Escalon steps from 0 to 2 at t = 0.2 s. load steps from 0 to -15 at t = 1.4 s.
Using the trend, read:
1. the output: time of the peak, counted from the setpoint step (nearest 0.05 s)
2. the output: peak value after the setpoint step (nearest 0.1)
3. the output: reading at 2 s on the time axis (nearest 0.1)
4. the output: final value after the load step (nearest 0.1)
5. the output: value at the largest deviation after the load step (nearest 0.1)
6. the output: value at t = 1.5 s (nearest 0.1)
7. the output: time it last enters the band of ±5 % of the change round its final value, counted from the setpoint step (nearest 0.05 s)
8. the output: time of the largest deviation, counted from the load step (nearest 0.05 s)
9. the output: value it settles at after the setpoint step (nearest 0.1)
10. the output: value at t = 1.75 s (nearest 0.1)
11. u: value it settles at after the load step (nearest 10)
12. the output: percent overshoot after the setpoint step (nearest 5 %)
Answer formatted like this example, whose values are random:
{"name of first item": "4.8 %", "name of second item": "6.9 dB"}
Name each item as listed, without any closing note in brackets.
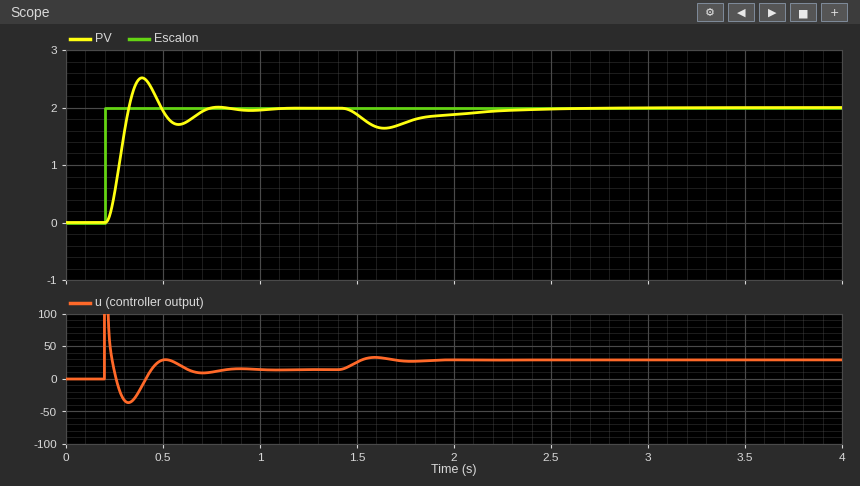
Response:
{"the output: time of the peak, counted from the setpoint step": "0.20 s", "the output: peak value after the setpoint step": "2.5", "the output: reading at 2 s on the time axis": "1.9", "the output: final value after the load step": "2.0", "the output: value at the largest deviation after the load step": "1.6", "the output: value at t = 1.5 s": "1.9", "the output: time it last enters the band of ±5 % of the change round its final value, counted from the setpoint step": "0.50 s", "the output: time of the largest deviation, counted from the load step": "0.25 s", "the output: value it settles at after the setpoint step": "2.0", "the output: value at t = 1.75 s": "1.7", "u: value it settles at after the load step": "30", "the output: percent overshoot after the setpoint step": "25 %"}
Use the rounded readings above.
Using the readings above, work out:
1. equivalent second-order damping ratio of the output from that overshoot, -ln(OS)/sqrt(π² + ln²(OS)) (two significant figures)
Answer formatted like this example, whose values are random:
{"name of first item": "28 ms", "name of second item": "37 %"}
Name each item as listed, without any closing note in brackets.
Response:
{"equivalent second-order damping ratio of the output from that overshoot, -ln(OS)/sqrt(π² + ln²(OS))": "0.40"}
